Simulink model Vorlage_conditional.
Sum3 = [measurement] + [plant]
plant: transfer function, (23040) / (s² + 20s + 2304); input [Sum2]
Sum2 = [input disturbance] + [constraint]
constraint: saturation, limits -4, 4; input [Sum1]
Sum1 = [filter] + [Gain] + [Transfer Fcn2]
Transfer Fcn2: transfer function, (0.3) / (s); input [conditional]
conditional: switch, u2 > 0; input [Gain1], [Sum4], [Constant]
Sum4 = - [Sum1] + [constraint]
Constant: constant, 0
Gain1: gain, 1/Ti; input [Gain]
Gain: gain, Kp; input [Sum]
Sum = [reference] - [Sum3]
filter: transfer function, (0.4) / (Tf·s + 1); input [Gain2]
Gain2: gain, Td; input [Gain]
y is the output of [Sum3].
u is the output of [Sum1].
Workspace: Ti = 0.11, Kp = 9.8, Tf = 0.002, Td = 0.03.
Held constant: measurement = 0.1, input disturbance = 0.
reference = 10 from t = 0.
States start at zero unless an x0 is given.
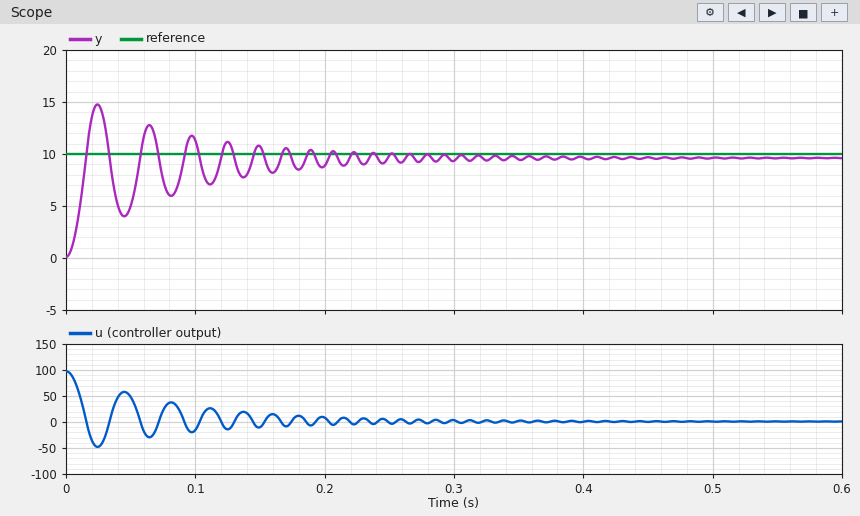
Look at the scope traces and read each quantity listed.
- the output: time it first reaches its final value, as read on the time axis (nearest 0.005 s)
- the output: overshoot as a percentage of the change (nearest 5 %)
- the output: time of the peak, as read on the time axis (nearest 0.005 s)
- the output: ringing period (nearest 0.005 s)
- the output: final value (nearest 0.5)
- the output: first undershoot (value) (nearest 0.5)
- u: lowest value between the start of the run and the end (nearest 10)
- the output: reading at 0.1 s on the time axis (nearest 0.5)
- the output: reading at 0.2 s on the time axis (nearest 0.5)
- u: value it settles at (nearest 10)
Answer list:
0.015 s
55 %
0.025 s
0.040 s
9.5
4.0
-50
11.5
9.0
0
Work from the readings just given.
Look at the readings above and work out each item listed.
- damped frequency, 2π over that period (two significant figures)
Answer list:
160 rad/s
